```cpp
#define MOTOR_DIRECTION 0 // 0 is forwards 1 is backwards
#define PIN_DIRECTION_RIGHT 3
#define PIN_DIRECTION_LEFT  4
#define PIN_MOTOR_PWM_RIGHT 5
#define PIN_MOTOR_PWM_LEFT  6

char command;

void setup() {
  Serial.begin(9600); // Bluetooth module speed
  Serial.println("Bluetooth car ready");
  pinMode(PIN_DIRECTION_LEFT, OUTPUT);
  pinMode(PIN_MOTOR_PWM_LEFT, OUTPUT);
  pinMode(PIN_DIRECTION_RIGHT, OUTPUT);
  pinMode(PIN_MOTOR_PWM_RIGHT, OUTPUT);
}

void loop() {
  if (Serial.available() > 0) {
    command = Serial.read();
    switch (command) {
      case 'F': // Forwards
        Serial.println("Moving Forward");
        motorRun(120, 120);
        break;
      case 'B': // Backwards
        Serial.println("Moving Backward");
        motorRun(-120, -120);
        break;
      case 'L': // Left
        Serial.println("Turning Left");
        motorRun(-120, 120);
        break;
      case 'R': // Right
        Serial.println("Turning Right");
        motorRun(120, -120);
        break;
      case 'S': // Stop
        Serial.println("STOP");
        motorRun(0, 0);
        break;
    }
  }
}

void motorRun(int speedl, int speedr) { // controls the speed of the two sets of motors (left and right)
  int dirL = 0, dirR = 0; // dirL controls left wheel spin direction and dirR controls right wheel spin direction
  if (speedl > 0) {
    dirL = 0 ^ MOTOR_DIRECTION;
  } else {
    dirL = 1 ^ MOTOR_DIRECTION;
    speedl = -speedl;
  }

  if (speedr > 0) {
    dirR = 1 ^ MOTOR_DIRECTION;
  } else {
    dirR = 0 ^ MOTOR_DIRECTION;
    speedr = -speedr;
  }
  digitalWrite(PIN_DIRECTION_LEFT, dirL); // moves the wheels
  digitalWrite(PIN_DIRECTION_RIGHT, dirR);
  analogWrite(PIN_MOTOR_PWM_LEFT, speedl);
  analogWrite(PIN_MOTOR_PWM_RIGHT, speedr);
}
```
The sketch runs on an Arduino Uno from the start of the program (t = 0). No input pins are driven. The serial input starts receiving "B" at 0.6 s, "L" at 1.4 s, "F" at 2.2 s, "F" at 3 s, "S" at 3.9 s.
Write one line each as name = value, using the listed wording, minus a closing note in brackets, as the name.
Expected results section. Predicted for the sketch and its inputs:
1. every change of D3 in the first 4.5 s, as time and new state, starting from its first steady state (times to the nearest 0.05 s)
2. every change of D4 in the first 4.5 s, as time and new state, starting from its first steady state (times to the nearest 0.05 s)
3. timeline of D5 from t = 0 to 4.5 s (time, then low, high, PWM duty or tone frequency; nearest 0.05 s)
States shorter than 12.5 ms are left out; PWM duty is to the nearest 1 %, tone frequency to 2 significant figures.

every change of D3 in the first 4.5 s, as time and new state, starting from its first steady state = 0 s low; 1.4 s high; 3.9 s low
every change of D4 in the first 4.5 s, as time and new state, starting from its first steady state = 0 s low; 0.6 s high; 2.2 s low; 3.9 s high
timeline of D5 from t = 0 to 4.5 s = 0 s low; 0.6 s PWM 47 %; 3.9 s low
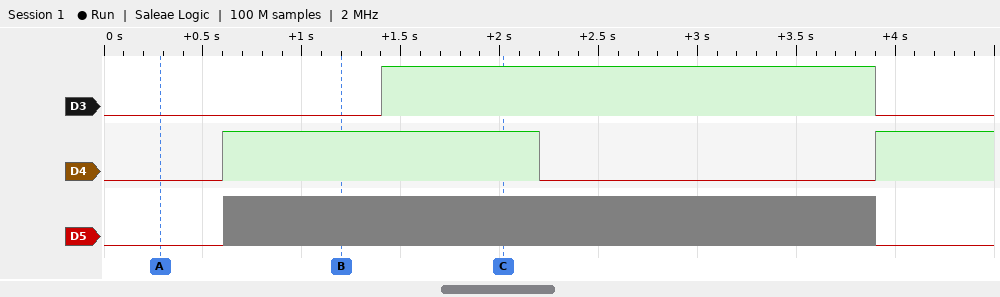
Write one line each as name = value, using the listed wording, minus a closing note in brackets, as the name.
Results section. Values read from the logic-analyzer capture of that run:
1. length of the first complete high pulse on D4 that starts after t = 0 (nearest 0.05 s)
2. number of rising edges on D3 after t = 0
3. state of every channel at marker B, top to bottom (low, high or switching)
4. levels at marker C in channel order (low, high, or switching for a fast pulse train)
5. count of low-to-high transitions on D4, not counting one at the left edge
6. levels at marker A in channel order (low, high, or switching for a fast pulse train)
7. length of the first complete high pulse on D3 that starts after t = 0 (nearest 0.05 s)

length of the first complete high pulse on D4 that starts after t = 0 = 1.60 s
number of rising edges on D3 after t = 0 = 1
state of every channel at marker B, top to bottom = D3 low, D4 high, D5 switching
levels at marker C in channel order = D3 high, D4 high, D5 switching
count of low-to-high transitions on D4, not counting one at the left edge = 2
levels at marker A in channel order = D3 low, D4 low, D5 low
length of the first complete high pulse on D3 that starts after t = 0 = 2.50 s
